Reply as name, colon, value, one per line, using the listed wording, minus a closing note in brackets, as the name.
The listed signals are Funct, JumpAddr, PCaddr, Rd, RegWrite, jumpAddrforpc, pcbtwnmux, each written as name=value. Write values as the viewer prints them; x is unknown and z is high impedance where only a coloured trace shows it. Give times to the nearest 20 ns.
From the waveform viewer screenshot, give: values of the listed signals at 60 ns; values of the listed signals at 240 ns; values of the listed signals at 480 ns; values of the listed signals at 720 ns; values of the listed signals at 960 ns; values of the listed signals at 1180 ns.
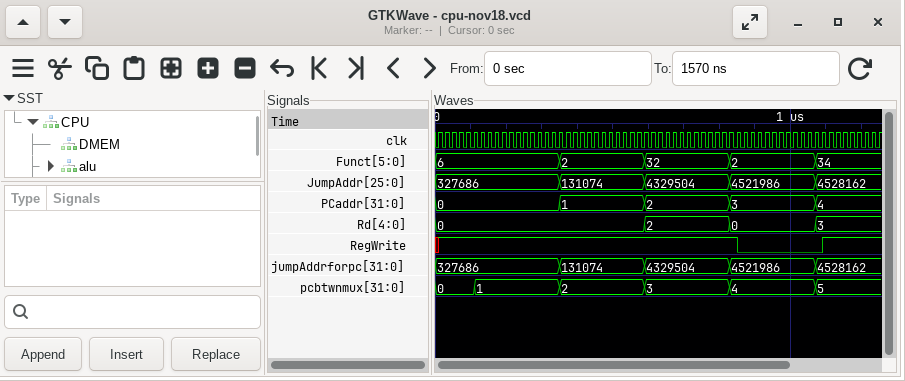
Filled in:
values of the listed signals at 60 ns: Funct=6, JumpAddr=327686, PCaddr=0, Rd=0, RegWrite=1, jumpAddrforpc=327686, pcbtwnmux=0
values of the listed signals at 240 ns: Funct=6, JumpAddr=327686, PCaddr=0, Rd=0, RegWrite=1, jumpAddrforpc=327686, pcbtwnmux=1
values of the listed signals at 480 ns: Funct=2, JumpAddr=131074, PCaddr=1, Rd=0, RegWrite=1, jumpAddrforpc=131074, pcbtwnmux=2
values of the listed signals at 720 ns: Funct=32, JumpAddr=4329504, PCaddr=2, Rd=2, RegWrite=1, jumpAddrforpc=4329504, pcbtwnmux=3
values of the listed signals at 960 ns: Funct=2, JumpAddr=4521986, PCaddr=3, Rd=0, RegWrite=0, jumpAddrforpc=4521986, pcbtwnmux=4
values of the listed signals at 1180 ns: Funct=34, JumpAddr=4528162, PCaddr=4, Rd=3, RegWrite=1, jumpAddrforpc=4528162, pcbtwnmux=5
